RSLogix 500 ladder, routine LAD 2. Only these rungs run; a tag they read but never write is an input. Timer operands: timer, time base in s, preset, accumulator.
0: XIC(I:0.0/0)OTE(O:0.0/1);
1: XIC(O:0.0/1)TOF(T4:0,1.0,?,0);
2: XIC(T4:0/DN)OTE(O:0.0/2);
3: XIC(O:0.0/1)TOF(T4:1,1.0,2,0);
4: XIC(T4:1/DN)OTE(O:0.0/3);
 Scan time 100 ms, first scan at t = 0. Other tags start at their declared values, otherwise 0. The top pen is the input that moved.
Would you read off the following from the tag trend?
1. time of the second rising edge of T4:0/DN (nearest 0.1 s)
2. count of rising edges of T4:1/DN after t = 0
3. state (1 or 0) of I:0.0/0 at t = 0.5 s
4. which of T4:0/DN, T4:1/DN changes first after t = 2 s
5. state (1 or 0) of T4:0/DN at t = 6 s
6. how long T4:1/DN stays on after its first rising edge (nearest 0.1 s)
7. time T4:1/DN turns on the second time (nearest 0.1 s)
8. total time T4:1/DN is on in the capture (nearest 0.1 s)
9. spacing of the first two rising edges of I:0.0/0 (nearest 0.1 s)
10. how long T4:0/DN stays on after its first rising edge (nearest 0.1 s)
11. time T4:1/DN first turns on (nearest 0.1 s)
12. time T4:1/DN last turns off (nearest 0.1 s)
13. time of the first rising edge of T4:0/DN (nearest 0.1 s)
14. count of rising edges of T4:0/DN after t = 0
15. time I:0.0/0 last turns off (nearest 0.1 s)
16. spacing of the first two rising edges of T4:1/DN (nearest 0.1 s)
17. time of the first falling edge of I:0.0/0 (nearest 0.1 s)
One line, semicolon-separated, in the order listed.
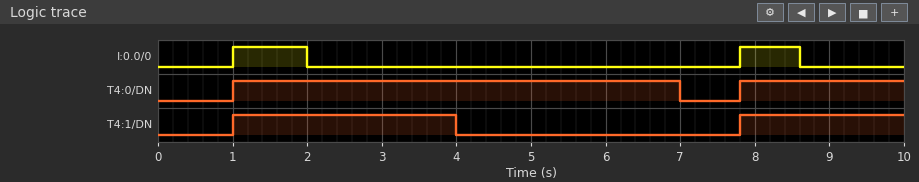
7.8 s; 2; 0; T4:1/DN; 1; 3.0 s; 7.8 s; 5.2 s; 6.8 s; 6.0 s; 1.0 s; 4.0 s; 1.0 s; 2; 8.6 s; 6.8 s; 2.0 s
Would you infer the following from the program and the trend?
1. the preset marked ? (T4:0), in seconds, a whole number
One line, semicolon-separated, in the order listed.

5 s
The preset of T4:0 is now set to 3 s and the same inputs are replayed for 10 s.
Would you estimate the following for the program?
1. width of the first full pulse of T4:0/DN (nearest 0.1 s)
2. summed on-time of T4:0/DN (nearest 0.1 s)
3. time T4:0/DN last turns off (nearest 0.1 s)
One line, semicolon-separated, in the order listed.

4.0 s; 6.2 s; 5.0 s
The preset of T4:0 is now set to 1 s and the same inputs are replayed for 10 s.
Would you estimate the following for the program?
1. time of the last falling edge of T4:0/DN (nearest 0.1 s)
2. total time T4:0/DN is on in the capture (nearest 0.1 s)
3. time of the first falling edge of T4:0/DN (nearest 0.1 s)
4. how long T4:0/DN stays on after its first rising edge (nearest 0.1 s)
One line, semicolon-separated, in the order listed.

9.6 s; 3.8 s; 3.0 s; 2.0 s
